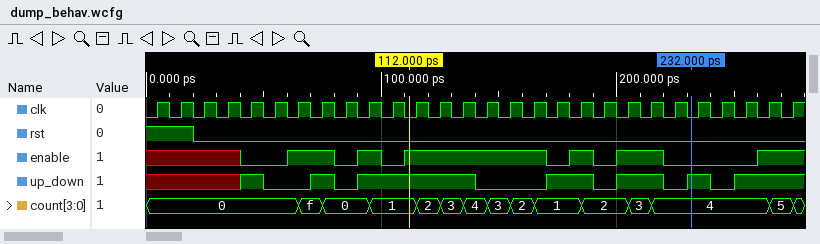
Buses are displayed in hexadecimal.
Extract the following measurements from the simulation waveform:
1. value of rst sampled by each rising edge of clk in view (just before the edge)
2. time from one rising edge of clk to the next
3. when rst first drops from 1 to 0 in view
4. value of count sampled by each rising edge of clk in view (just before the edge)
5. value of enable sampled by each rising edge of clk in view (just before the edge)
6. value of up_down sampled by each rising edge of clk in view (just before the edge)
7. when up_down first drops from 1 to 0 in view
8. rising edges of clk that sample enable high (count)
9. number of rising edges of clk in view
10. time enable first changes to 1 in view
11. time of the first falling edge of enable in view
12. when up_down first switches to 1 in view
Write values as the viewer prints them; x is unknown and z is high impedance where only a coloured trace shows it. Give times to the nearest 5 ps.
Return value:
1 1 0 0 0 0 0 0 0 0 0 0 0 0 0 0 0 0 0 0 0 0 0 0 0 0 0 0
10 ps
20 ps
0, 0, 0, 0, 0, 0, 0, f, 0, 0, 1, 1, 2, 3, 4, 3, 2, 1, 1, 2, 2, 3, 4, 4, 4, 4, 4, 5
x x x x 0 0 1 1 0 1 0 1 1 1 1 1 1 0 1 0 1 1 0 0 0 0 1 1
x x x x 1 0 0 1 0 1 1 1 1 1 0 0 0 1 1 0 1 1 0 1 0 1 1 1
50 ps
14
28
60 ps
80 ps
40 ps
